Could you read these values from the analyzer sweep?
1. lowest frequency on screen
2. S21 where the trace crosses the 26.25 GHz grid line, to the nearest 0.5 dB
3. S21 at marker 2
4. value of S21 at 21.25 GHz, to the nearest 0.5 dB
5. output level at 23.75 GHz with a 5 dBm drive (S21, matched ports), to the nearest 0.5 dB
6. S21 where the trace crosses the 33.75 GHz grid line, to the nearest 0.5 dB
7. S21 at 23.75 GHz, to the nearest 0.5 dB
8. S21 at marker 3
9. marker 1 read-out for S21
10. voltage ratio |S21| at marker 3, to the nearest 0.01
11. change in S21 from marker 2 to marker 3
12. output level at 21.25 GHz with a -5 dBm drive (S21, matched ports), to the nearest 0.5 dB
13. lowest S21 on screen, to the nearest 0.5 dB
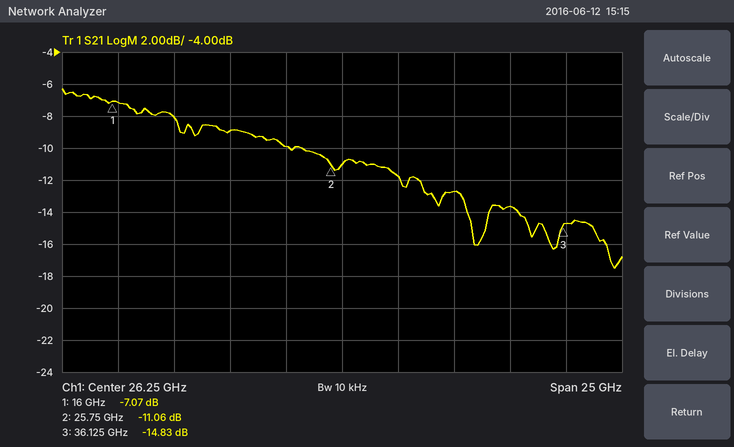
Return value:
13.75 GHz
-11.0 dB
-11.06 dB
-9.0 dB
-5.0 dBm
-13.5 dB
-10.0 dB
-14.83 dB
-7.07 dB
0.18
-3.77 dB
-14.0 dBm
-17.5 dB
